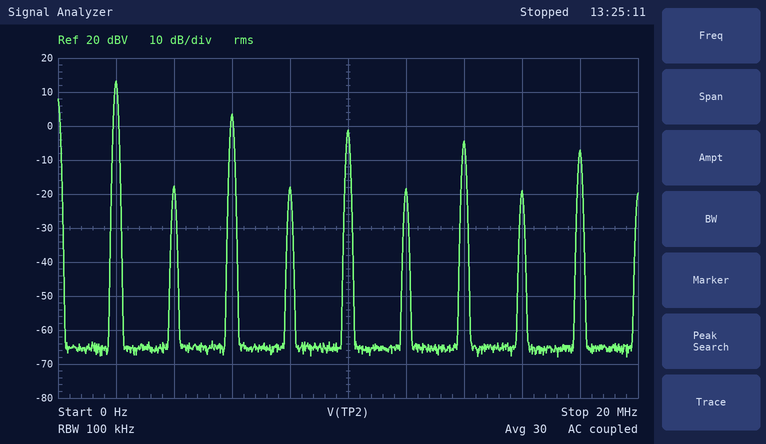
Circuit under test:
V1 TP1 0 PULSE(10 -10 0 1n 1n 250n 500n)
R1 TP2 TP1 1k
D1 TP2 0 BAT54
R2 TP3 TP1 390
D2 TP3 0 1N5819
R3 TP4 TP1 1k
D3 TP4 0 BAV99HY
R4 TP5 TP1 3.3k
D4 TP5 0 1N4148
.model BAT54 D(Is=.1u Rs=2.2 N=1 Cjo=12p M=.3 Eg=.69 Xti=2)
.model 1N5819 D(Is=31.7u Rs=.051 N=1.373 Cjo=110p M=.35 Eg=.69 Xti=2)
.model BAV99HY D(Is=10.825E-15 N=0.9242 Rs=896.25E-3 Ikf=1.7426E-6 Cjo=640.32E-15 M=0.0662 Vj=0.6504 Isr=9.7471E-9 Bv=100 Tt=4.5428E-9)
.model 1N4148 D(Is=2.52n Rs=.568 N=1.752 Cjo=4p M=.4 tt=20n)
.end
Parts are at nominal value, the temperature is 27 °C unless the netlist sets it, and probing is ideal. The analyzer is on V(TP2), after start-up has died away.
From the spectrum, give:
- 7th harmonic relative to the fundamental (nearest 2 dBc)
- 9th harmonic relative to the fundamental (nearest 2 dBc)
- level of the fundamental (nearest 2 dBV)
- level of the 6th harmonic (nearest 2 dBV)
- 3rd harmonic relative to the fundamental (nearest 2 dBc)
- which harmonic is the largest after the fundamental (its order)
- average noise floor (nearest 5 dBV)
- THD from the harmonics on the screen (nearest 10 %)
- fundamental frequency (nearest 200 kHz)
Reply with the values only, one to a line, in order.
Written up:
-18 dBc
-20 dBc
14 dBV
-18 dBV
-10 dBc
3
-65 dBV
40 %
2.0 MHz
